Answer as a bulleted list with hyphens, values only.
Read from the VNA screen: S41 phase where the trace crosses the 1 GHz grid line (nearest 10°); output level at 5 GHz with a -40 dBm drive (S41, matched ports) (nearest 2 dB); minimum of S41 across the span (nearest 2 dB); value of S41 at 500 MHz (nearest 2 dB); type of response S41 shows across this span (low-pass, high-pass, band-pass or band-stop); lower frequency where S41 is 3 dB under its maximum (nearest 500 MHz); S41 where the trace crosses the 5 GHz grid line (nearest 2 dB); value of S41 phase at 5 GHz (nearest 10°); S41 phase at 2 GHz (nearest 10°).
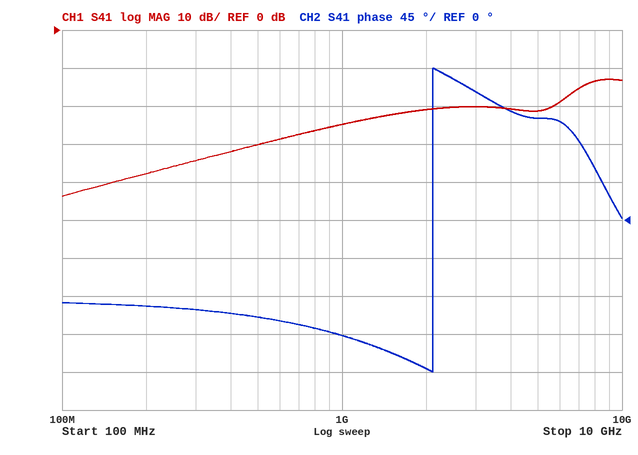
- -140°
- -62 dBm
- -44 dB
- -30 dB
- high-pass
- 7.0 GHz
- -22 dB
- 120°
- -180°
